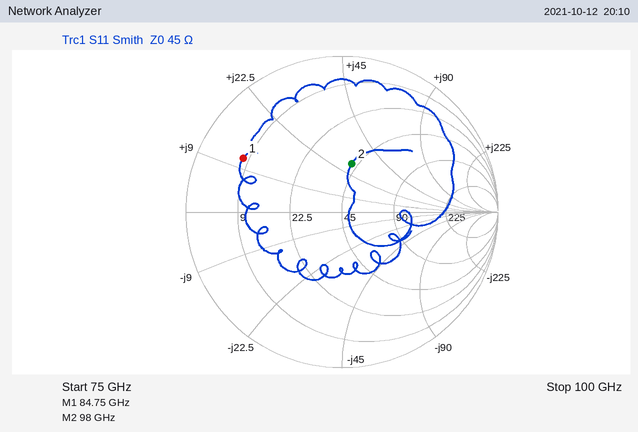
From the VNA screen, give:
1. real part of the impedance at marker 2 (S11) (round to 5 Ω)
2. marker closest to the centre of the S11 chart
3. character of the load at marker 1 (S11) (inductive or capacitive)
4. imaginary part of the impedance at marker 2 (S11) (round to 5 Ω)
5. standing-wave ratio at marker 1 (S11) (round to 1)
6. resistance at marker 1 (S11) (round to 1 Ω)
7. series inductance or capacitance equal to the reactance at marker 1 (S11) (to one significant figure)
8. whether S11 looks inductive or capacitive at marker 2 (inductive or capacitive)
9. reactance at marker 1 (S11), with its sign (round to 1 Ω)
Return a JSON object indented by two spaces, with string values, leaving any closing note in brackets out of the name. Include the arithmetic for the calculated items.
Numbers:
{
  "real part of the impedance at marker 2 (S11)": "40 Ω",
  "marker closest to the centre of the S11 chart": "marker 2",
  "character of the load at marker 1 (S11)": "inductive",
  "imaginary part of the impedance at marker 2 (S11)": "+30 Ω",
  "standing-wave ratio at marker 1 (S11)": "6",
  "resistance at marker 1 (S11)": "8 Ω",
  "series inductance or capacitance equal to the reactance at marker 1 (S11)": "L = 11 Ω/(2π × 84.75 GHz) ≈ 20.7 pH, so 20 pH to one significant figure",
  "whether S11 looks inductive or capacitive at marker 2": "inductive",
  "reactance at marker 1 (S11), with its sign": "+11 Ω"
}
